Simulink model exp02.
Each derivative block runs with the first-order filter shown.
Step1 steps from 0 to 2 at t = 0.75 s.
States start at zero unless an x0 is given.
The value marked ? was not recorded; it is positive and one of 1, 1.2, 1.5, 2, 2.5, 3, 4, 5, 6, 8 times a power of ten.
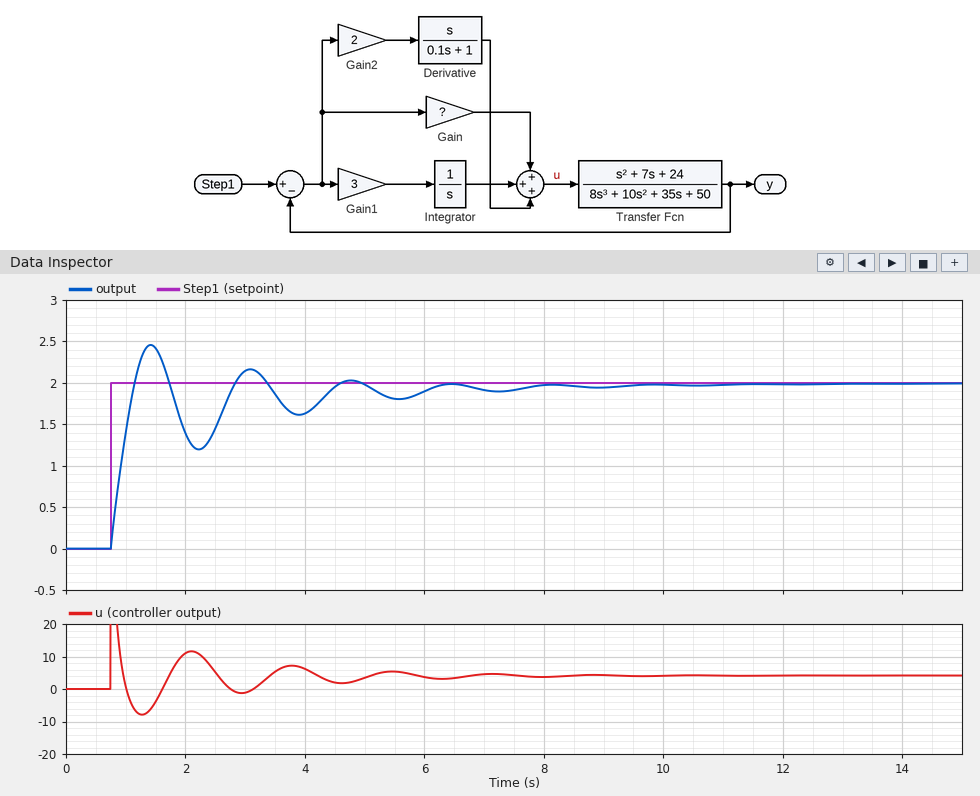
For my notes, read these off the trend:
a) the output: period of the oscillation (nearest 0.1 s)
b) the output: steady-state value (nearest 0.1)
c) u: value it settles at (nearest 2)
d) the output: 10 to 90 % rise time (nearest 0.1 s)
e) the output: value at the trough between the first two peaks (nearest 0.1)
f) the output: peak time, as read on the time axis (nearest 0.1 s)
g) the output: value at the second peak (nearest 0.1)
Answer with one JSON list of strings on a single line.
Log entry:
["1.7 s", "2.0", "4", "0.3 s", "1.2", "1.4 s", "2.2"]
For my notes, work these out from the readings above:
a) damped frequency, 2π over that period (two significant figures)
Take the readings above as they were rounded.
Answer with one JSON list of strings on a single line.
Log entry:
["3.7 rad/s"]
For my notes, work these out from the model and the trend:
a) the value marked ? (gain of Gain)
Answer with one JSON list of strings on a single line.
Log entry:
["10"]
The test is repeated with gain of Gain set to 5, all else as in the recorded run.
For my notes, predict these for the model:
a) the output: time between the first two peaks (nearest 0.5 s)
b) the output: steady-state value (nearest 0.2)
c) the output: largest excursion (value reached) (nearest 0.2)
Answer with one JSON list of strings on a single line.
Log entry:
["2.0 s", "2.0", "2.2"]
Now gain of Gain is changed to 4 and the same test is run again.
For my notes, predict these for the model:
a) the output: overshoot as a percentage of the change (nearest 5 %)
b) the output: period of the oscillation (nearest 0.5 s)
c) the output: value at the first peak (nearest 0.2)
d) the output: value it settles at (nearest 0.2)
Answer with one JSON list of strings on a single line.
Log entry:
["10 %", "2.0 s", "2.2", "2.0"]
